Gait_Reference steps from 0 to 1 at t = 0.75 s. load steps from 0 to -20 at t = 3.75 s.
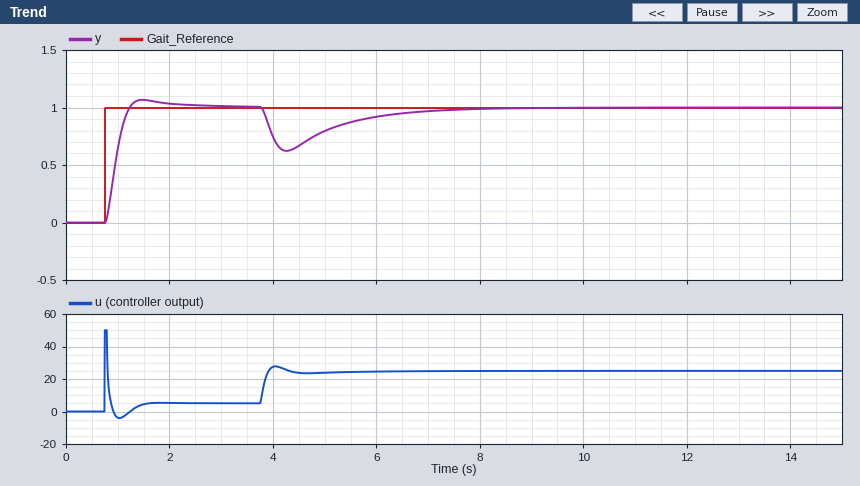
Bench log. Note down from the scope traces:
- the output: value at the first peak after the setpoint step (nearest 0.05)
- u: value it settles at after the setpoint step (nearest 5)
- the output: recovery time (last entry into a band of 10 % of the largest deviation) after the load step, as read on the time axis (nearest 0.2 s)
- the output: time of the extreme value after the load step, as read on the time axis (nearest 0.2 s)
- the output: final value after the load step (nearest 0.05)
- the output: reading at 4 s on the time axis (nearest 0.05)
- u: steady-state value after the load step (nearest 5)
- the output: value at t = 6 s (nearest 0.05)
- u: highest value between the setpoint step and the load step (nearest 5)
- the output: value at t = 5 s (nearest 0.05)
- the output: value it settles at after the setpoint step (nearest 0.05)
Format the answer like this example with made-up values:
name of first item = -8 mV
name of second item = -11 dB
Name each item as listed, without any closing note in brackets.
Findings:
the output: value at the first peak after the setpoint step = 1.05
u: value it settles at after the setpoint step = 5
the output: recovery time (last entry into a band of 10 % of the largest deviation) after the load step, as read on the time axis = 6.8 s
the output: time of the extreme value after the load step, as read on the time axis = 4.2 s
the output: final value after the load step = 1.00
the output: reading at 4 s on the time axis = 0.75
u: steady-state value after the load step = 25
the output: value at t = 6 s = 0.90
u: highest value between the setpoint step and the load step = 50
the output: value at t = 5 s = 0.80
the output: value it settles at after the setpoint step = 1.00
